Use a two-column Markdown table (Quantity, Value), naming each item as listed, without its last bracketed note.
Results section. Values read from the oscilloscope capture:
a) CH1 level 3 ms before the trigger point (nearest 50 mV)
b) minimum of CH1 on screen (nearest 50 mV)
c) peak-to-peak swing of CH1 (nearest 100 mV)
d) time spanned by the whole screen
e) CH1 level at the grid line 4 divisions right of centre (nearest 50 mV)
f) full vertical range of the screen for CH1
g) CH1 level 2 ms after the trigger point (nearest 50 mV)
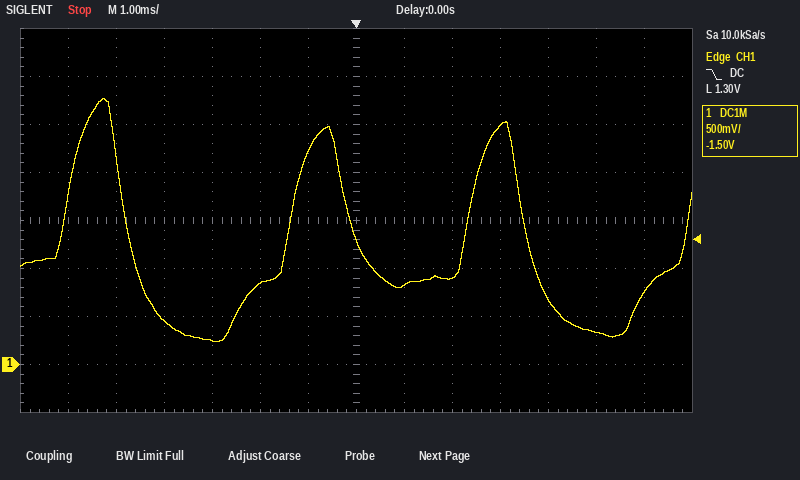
| Quantity | Value |
|---|---|
| CH1 level 3 ms before the trigger point | 250 mV |
| minimum of CH1 on screen | 250 mV |
| peak-to-peak swing of CH1 | 2.50 V |
| time spanned by the whole screen | 14 ms |
| CH1 level at the grid line 4 divisions right of centre | 700 mV |
| full vertical range of the screen for CH1 | 4 V |
| CH1 level 2 ms after the trigger point | 900 mV |
